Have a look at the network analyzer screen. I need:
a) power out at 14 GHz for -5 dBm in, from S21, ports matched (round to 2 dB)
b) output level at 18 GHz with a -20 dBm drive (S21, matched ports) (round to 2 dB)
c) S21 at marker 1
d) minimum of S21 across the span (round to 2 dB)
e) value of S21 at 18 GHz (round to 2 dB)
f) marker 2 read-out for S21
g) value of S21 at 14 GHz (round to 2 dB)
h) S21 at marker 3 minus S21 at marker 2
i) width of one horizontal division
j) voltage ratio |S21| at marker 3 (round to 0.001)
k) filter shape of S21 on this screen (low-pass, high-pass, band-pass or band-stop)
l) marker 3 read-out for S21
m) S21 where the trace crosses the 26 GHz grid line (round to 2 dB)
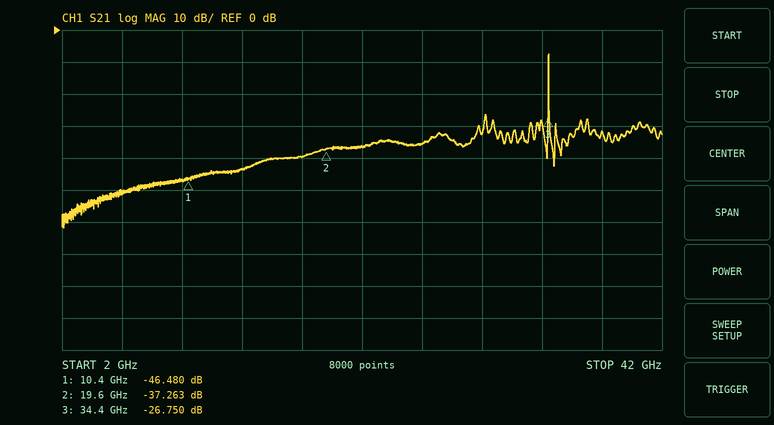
-48 dBm
-60 dBm
-46.480 dB
-62 dB
-40 dB
-37.263 dB
-44 dB
10.513 dB
4 GHz
0.046
band-pass
-26.750 dB
-36 dB
